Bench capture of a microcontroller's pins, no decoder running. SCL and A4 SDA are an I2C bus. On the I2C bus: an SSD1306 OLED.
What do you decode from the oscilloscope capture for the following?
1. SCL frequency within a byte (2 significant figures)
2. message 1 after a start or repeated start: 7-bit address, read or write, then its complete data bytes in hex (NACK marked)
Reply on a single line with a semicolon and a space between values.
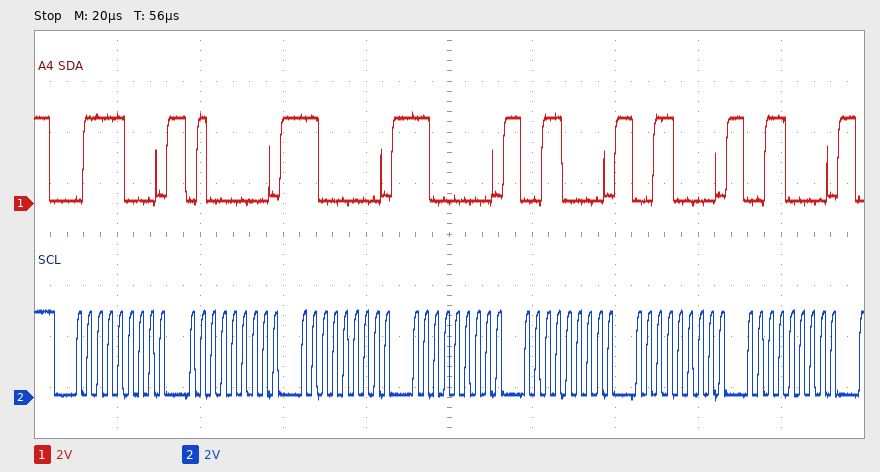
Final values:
400 kHz; 0x3C write: 40 C0 C0 30 30 30
